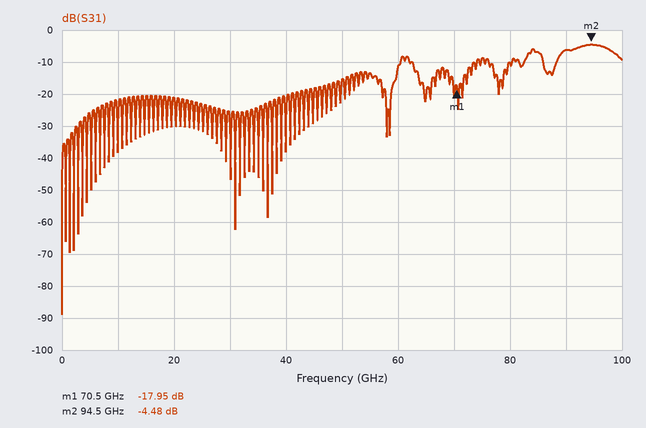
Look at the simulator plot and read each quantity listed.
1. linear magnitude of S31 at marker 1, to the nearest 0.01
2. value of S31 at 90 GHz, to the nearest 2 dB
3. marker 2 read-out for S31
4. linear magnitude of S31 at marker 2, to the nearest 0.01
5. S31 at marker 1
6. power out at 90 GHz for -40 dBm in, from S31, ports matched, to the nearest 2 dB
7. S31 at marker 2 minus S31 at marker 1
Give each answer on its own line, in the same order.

0.13
-6 dB
-4.48 dB
0.60
-17.95 dB
-46 dBm
13.47 dB
